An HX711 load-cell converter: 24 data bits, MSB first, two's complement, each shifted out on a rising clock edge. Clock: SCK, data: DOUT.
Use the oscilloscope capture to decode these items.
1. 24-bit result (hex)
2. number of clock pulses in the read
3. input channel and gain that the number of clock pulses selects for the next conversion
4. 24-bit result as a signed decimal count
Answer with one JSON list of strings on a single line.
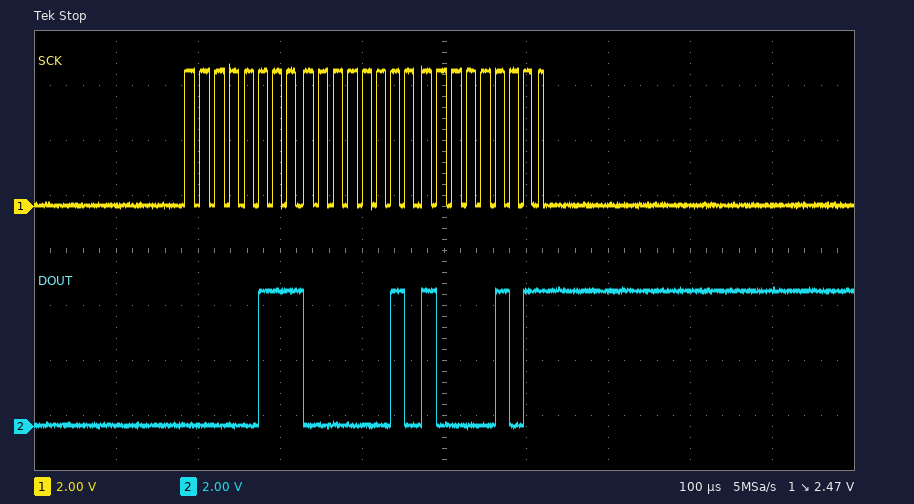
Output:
["0x070285", "25", "channel A, gain 128", "459397"]
